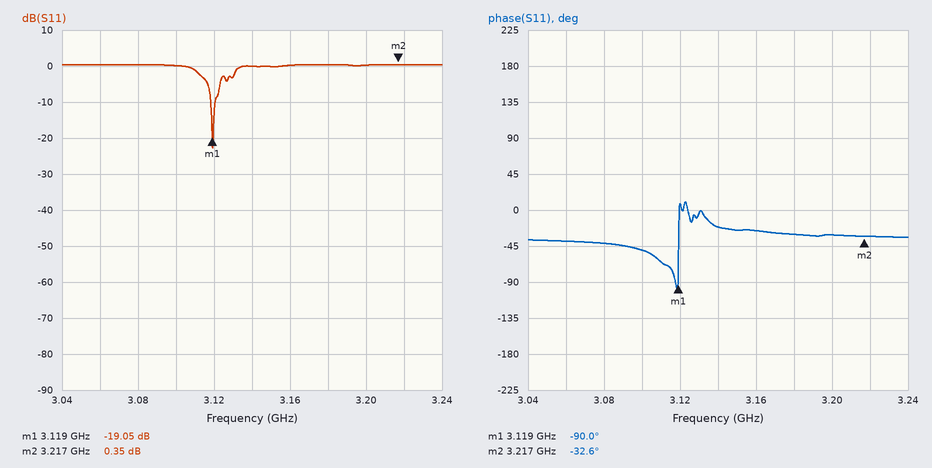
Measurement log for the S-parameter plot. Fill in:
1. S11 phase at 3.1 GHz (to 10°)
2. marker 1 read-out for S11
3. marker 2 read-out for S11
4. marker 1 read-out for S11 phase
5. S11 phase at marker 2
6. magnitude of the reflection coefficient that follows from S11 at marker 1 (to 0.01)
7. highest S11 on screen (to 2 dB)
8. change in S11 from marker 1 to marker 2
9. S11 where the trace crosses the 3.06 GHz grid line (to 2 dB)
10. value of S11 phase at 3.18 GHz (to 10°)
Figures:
-50°
-19.05 dB
0.35 dB
-90.0°
-32.6°
0.11
0 dB
19.40 dB
0 dB
-30°
